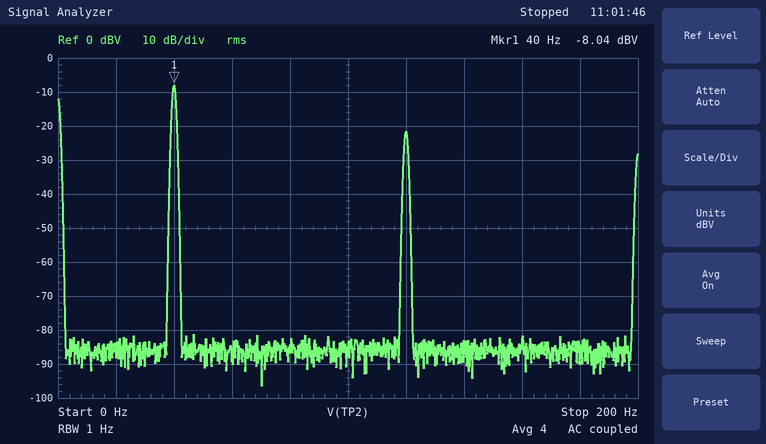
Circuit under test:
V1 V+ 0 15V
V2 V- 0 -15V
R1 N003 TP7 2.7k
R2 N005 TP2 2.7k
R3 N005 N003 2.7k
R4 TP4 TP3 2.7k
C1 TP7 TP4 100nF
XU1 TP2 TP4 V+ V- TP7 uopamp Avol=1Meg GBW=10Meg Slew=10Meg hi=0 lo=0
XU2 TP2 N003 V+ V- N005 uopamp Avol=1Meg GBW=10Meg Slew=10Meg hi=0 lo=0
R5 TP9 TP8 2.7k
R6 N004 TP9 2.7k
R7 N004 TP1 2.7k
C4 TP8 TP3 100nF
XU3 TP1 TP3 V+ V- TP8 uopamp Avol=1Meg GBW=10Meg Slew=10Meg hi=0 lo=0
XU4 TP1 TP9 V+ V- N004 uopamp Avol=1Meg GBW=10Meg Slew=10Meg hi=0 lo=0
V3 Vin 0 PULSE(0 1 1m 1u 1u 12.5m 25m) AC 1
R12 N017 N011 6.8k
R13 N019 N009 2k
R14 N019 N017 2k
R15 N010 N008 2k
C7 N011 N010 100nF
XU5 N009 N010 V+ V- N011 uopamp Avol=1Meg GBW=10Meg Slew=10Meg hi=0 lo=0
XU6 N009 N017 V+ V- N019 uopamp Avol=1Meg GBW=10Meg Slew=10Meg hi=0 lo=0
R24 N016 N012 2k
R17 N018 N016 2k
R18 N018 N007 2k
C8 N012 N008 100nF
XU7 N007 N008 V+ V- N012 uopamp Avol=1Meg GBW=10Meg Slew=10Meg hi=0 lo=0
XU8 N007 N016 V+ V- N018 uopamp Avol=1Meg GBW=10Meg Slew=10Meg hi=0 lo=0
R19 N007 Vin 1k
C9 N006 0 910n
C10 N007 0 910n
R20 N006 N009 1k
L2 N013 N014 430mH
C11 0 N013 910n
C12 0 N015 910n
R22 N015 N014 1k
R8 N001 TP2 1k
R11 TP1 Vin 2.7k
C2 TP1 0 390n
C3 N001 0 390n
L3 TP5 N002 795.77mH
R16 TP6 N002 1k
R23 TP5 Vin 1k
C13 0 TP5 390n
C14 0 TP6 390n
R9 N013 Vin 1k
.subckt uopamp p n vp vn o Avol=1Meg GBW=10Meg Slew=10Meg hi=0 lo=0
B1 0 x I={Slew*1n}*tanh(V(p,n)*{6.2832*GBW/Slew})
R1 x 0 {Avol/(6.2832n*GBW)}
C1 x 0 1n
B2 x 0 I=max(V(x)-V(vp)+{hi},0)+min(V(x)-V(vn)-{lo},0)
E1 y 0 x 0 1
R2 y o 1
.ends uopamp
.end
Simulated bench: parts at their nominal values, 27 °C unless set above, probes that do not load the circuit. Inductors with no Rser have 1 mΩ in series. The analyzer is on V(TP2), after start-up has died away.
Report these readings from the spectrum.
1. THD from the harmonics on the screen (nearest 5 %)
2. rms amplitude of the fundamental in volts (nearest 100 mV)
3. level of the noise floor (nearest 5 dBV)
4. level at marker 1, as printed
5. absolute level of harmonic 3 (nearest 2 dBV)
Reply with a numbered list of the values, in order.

1. 20 %
2. 400 mV
3. -85 dBV
4. -8.04 dBV
5. -22 dBV
